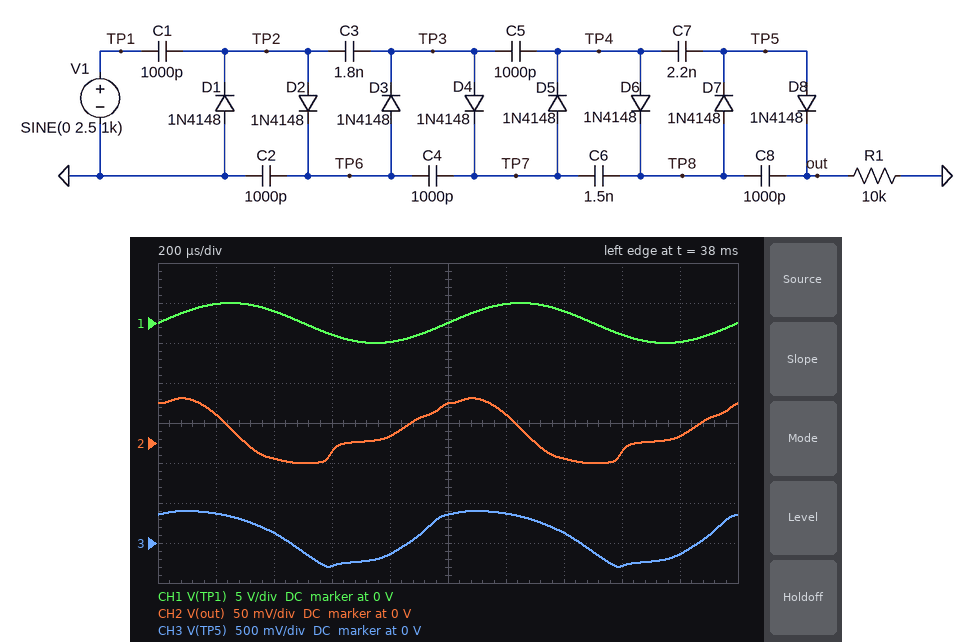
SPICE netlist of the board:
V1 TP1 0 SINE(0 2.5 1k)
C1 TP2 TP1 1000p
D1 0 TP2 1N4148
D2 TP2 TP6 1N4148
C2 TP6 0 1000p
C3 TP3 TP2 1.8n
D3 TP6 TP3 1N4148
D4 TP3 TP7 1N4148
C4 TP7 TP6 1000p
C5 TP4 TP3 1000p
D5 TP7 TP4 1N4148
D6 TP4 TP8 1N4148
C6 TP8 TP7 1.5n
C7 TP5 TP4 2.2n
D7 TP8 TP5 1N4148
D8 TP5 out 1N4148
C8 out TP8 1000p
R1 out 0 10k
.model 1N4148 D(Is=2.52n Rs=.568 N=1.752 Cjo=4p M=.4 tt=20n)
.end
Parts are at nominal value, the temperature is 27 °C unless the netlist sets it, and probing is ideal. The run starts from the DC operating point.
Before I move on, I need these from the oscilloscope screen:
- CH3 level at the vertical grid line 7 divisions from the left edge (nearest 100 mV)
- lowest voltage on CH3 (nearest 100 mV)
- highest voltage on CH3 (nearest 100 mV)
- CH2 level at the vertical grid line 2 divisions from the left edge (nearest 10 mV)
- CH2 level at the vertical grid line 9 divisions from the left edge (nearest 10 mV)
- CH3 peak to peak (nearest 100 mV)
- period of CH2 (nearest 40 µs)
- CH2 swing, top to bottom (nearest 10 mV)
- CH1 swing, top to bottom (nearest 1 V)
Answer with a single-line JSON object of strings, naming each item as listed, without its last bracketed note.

{"CH3 level at the vertical grid line 7 divisions from the left edge": "100 mV", "lowest voltage on CH3": "-300 mV", "highest voltage on CH3": "400 mV", "CH2 level at the vertical grid line 2 divisions from the left edge": "-20 mV", "CH2 level at the vertical grid line 9 divisions from the left edge": "10 mV", "CH3 peak to peak": "700 mV", "period of CH2": "1.00 ms", "CH2 swing, top to bottom": "80 mV", "CH1 swing, top to bottom": "5 V"}
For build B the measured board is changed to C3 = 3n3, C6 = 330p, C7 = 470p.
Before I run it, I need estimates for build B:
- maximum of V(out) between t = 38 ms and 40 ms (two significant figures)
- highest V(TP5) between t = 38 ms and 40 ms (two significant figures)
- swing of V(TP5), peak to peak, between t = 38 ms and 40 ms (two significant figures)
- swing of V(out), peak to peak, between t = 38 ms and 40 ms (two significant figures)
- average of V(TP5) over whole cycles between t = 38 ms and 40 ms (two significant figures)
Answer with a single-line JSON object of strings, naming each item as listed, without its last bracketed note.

{"maximum of V(out) between t = 38 ms and 40 ms": "51 mV", "highest V(TP5) between t = 38 ms and 40 ms": "390 mV", "swing of V(TP5), peak to peak, between t = 38 ms and 40 ms": "560 mV", "swing of V(out), peak to peak, between t = 38 ms and 40 ms": "72 mV", "average of V(TP5) over whole cycles between t = 38 ms and 40 ms": "180 mV"}
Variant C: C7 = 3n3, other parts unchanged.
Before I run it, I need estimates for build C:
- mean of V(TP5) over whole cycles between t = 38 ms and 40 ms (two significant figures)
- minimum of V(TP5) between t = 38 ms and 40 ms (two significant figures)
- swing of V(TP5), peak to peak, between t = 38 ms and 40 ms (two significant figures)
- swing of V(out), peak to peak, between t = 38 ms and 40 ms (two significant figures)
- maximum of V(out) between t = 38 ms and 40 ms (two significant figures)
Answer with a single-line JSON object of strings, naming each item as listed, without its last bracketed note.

{"mean of V(TP5) over whole cycles between t = 38 ms and 40 ms": "69 mV", "minimum of V(TP5) between t = 38 ms and 40 ms": "-320 mV", "swing of V(TP5), peak to peak, between t = 38 ms and 40 ms": "720 mV", "swing of V(out), peak to peak, between t = 38 ms and 40 ms": "84 mV", "maximum of V(out) between t = 38 ms and 40 ms": "58 mV"}
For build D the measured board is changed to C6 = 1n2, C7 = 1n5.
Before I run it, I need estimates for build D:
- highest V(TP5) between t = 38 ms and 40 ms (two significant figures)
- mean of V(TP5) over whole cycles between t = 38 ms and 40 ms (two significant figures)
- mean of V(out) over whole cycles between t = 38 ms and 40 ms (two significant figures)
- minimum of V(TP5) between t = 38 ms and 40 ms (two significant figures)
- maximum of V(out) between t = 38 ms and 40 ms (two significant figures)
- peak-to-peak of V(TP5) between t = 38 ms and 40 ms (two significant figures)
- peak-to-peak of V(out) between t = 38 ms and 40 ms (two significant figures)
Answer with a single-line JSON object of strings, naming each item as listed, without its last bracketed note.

{"highest V(TP5) between t = 38 ms and 40 ms": "390 mV", "mean of V(TP5) over whole cycles between t = 38 ms and 40 ms": "110 mV", "mean of V(out) over whole cycles between t = 38 ms and 40 ms": "12 mV", "minimum of V(TP5) between t = 38 ms and 40 ms": "-270 mV", "maximum of V(out) between t = 38 ms and 40 ms": "52 mV", "peak-to-peak of V(TP5) between t = 38 ms and 40 ms": "660 mV", "peak-to-peak of V(out) between t = 38 ms and 40 ms": "77 mV"}
